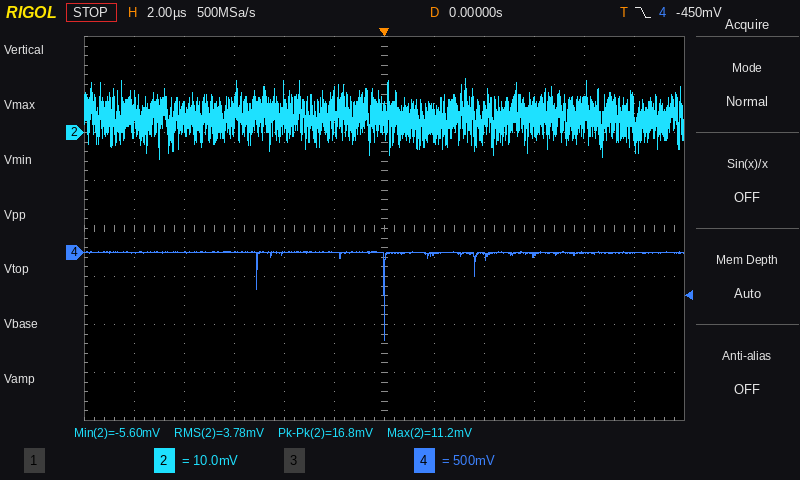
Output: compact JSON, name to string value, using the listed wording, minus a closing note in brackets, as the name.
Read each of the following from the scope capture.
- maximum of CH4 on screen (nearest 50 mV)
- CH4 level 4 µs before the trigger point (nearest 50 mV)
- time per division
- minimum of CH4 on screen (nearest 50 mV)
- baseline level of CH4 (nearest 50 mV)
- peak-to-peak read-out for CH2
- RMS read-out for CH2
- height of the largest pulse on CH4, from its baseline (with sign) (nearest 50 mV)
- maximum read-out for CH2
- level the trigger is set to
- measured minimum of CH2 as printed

{"maximum of CH4 on screen": "0 mV", "CH4 level 4 µs before the trigger point": "0 mV", "time per division": "2 µs", "minimum of CH4 on screen": "-900 mV", "baseline level of CH4": "0 mV", "peak-to-peak read-out for CH2": "16.8 mV", "RMS read-out for CH2": "3.78 mV", "height of the largest pulse on CH4, from its baseline (with sign)": "-900 mV", "maximum read-out for CH2": "11.2 mV", "level the trigger is set to": "-450 mV", "measured minimum of CH2 as printed": "-5.60 mV"}
